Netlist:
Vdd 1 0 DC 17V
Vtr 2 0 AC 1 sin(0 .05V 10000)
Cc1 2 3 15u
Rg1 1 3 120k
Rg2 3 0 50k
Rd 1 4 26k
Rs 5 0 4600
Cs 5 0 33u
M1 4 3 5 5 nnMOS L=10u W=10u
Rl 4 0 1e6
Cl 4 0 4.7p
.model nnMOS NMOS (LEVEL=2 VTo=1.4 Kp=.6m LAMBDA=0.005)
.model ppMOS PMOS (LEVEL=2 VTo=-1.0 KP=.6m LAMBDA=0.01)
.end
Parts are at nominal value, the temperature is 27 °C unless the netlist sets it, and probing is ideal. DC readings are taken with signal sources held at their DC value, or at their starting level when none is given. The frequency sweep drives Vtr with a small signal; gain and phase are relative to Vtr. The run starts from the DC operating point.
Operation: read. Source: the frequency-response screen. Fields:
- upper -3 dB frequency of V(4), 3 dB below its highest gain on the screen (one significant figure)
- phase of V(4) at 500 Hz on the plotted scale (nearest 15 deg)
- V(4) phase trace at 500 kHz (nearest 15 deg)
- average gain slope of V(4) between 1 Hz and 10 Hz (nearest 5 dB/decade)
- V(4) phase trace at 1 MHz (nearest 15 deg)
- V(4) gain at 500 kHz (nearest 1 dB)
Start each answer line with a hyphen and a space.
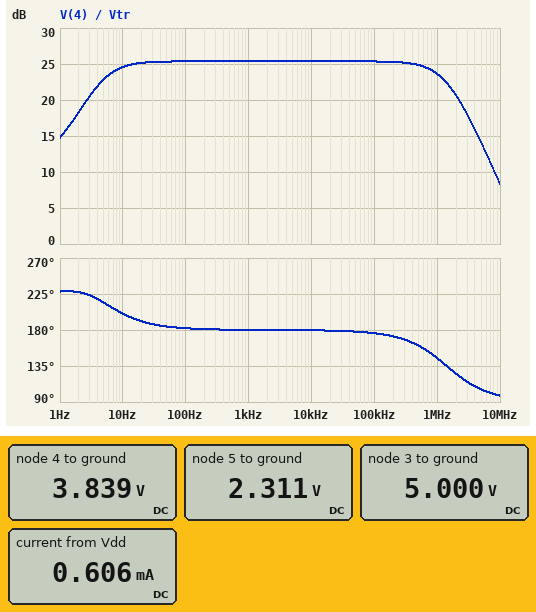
- 1 MHz
- 180 deg
- 165 deg
- 10 dB/decade
- 150 deg
- 25 dB
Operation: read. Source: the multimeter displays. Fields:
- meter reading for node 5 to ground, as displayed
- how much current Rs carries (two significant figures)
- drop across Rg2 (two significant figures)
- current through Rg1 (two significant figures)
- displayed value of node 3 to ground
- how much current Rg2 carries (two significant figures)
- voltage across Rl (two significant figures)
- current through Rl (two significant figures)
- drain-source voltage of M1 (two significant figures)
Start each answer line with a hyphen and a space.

- 2.311 V
- 500 µA
- 5.0 V
- 100 µA
- 5.000 V
- 100 µA
- 3.8 V
- 3.8 µA
- 1.5 V
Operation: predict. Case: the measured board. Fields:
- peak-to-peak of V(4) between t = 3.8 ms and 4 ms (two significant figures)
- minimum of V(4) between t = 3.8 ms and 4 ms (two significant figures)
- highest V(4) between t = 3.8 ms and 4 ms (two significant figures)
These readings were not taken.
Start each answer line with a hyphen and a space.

- 1.4 V
- 3.4 V
- 4.7 V
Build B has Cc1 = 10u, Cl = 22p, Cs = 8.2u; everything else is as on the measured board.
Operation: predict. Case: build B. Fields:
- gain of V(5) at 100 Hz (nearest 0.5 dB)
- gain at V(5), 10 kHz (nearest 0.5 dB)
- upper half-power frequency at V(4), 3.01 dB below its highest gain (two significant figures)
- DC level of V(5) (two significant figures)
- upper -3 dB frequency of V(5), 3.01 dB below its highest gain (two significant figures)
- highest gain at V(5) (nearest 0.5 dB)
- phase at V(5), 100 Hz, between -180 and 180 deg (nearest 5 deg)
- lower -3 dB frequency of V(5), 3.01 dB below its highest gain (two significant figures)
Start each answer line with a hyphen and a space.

- -17.0 dB
- -57.0 dB
- 300 kHz
- 2.3 V
- 19 Hz
- -2.5 dB
- -80 deg
- 430 mHz
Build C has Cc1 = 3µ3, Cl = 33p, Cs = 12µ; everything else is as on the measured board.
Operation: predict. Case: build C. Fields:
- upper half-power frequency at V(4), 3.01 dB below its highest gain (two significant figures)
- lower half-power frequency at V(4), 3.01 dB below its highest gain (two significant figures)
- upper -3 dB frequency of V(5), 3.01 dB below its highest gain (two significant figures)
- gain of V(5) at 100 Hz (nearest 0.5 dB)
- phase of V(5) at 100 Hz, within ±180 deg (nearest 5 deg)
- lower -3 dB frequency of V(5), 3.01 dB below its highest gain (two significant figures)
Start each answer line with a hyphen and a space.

- 200 kHz
- 12 Hz
- 15 Hz
- -20.5 dB
- -80 deg
- 1.1 Hz
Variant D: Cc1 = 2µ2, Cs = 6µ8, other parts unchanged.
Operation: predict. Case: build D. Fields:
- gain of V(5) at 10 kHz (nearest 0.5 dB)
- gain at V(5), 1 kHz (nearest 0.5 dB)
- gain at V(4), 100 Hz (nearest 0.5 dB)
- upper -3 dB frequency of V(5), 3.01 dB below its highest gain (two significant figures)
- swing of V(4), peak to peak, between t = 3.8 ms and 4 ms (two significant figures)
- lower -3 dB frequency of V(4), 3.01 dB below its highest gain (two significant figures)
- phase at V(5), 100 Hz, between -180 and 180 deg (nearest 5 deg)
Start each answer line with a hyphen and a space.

- -55.5 dB
- -35.5 dB
- 25.0 dB
- 26 Hz
- 1.3 V
- 21 Hz
- -75 deg
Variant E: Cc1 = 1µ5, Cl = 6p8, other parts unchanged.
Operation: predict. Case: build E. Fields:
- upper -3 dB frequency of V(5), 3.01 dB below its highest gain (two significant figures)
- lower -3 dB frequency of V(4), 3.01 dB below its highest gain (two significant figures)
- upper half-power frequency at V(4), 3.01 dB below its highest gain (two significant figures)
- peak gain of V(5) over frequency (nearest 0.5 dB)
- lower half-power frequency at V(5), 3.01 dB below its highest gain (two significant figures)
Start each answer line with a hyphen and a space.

- 9.1 Hz
- 5.8 Hz
- 980 kHz
- -6.5 dB
- 1.5 Hz
